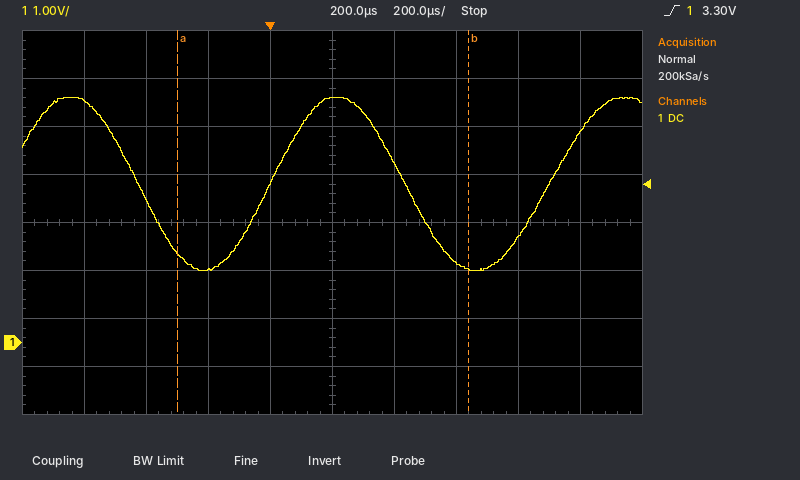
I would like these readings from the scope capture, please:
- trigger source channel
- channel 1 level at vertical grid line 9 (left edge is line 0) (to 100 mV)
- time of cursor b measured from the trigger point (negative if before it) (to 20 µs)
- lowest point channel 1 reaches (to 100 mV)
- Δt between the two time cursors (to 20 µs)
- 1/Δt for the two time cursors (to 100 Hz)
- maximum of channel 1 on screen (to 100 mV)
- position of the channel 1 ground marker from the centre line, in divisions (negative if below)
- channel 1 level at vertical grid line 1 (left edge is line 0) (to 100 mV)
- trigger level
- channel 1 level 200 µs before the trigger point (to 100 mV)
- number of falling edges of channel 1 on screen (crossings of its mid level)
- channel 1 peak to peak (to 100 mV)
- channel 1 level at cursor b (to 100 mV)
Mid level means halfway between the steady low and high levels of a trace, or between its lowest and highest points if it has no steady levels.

channel 1
4.4 V
+640 µs
1.5 V
940 µs
1.1 kHz
5.1 V
-2.5 div
5.0 V
3.30 V
1.5 V
2
3.6 V
1.5 V
